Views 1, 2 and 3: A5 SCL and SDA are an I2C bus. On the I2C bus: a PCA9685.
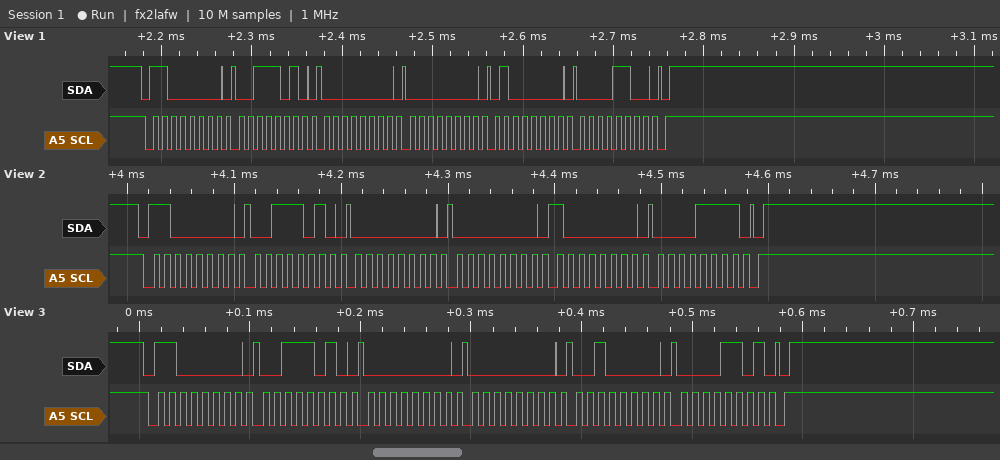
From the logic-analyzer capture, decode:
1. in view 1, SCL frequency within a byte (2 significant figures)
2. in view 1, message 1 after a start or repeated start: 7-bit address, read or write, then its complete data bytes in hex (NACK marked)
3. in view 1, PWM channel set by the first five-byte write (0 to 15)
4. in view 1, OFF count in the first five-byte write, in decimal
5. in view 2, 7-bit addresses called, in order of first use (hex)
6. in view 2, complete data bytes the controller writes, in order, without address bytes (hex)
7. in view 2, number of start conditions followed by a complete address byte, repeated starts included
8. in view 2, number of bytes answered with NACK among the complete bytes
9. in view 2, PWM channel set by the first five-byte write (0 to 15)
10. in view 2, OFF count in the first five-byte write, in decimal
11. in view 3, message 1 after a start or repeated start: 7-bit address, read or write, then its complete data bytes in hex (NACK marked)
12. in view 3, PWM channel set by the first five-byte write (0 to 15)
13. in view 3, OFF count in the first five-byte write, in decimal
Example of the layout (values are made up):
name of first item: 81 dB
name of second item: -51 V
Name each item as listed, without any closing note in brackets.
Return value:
in view 1, SCL frequency within a byte: 100 kHz
in view 1, message 1 after a start or repeated start: 7-bit address, read or write, then its complete data bytes in hex: 0x60 write: 3A 00 00 40 0C
in view 1, PWM channel set by the first five-byte write: 13
in view 1, OFF count in the first five-byte write, in decimal: 3136
in view 2, 7-bit addresses called, in order of first use: 0x60
in view 2, complete data bytes the controller writes, in order, without address bytes: 3A 00 00 80 0F
in view 2, number of start conditions followed by a complete address byte, repeated starts included: 1
in view 2, number of bytes answered with NACK among the complete bytes: 0
in view 2, PWM channel set by the first five-byte write: 13
in view 2, OFF count in the first five-byte write, in decimal: 3968
in view 3, message 1 after a start or repeated start: 7-bit address, read or write, then its complete data bytes in hex: 0x60 write: 3A 00 00 20 0D
in view 3, PWM channel set by the first five-byte write: 13
in view 3, OFF count in the first five-byte write, in decimal: 3360
